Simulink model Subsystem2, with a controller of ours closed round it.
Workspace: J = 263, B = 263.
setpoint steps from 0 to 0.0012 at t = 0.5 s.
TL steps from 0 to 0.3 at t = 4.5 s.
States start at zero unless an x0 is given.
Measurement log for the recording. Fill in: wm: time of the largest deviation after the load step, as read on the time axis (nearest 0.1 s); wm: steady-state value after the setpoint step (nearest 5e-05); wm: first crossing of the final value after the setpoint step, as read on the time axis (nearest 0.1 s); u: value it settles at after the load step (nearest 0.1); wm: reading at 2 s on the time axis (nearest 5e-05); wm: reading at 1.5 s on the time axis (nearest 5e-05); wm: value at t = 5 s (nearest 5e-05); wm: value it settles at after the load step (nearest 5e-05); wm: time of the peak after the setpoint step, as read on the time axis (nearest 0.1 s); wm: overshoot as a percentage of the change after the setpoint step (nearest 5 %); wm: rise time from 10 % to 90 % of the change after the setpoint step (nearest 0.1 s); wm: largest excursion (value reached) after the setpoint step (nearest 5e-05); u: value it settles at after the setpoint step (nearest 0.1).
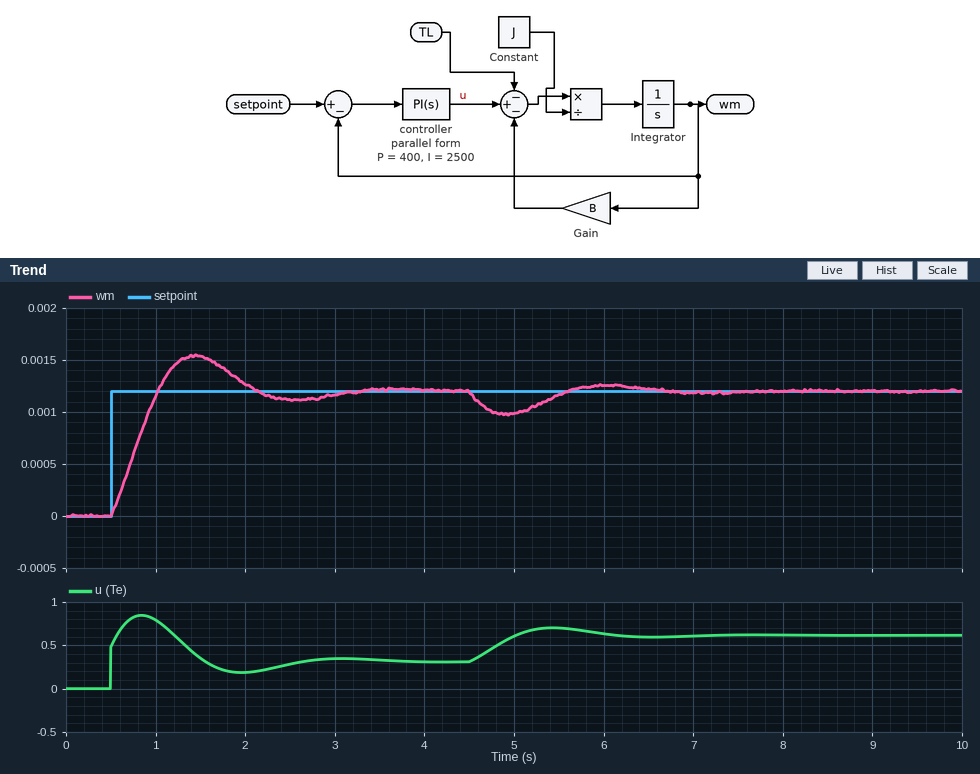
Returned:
4.9 s
0.00120
1.0 s
0.6
0.00125
0.00155
0.00100
0.00120
1.4 s
30 %
0.4 s
0.00155
0.3
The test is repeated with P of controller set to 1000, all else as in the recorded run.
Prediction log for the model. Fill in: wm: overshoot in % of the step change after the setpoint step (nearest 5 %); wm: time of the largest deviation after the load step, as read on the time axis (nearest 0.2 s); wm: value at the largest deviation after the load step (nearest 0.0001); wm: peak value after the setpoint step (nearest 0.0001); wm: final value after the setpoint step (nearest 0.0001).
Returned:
10 %
4.8 s
0.0010
0.0013
0.0012
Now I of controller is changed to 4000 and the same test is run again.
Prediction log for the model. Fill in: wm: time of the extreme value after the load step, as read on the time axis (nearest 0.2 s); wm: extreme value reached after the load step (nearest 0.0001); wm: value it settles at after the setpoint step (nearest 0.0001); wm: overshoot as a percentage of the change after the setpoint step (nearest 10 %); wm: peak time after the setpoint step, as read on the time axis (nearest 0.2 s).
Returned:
4.8 s
0.0010
0.0012
40 %
1.2 s
